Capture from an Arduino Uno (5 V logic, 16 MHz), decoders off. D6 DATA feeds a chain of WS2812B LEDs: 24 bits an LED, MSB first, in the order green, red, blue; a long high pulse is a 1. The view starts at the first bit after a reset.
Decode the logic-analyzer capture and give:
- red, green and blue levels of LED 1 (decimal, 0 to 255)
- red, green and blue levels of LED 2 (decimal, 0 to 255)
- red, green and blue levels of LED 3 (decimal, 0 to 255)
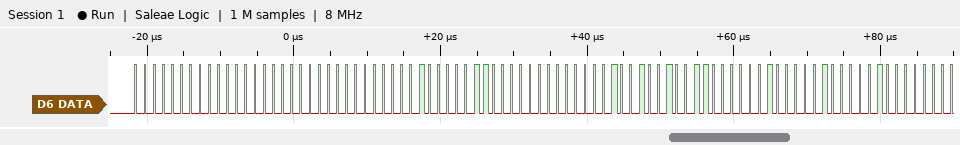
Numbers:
0, 0, 0
6, 1, 0
38, 9, 4
